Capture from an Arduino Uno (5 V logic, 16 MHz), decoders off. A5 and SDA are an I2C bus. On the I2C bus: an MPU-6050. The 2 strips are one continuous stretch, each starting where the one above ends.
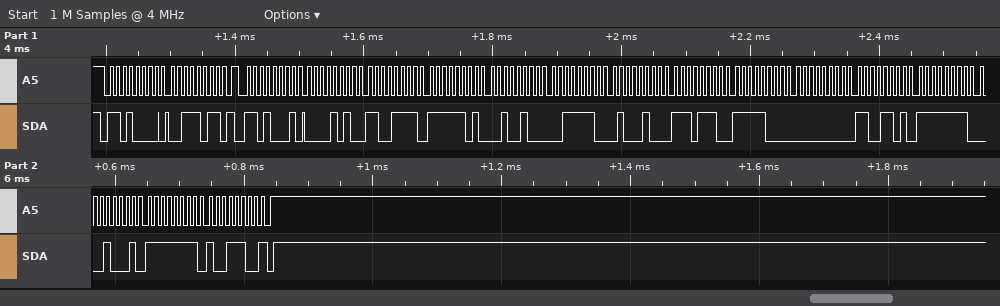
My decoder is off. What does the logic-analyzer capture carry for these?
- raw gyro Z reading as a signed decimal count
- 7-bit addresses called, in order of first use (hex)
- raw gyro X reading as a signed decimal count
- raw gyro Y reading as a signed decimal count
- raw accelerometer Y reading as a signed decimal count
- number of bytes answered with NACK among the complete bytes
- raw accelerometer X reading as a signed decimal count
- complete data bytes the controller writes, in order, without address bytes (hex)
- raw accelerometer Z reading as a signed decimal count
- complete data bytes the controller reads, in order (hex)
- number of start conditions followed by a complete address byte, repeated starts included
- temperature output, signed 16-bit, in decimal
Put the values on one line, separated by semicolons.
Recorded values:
-100; 0x68; 205; -239; -732; 1; 2767; 3B; 15940; 0A CF FD 24 3E 44 EE F8 00 CD FF 11 FF 9C; 2; -4360
